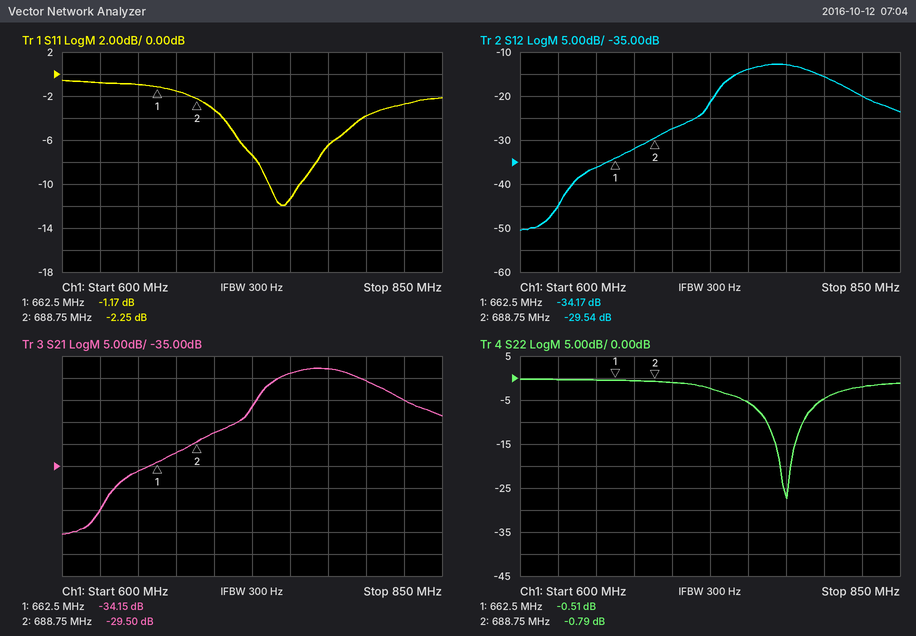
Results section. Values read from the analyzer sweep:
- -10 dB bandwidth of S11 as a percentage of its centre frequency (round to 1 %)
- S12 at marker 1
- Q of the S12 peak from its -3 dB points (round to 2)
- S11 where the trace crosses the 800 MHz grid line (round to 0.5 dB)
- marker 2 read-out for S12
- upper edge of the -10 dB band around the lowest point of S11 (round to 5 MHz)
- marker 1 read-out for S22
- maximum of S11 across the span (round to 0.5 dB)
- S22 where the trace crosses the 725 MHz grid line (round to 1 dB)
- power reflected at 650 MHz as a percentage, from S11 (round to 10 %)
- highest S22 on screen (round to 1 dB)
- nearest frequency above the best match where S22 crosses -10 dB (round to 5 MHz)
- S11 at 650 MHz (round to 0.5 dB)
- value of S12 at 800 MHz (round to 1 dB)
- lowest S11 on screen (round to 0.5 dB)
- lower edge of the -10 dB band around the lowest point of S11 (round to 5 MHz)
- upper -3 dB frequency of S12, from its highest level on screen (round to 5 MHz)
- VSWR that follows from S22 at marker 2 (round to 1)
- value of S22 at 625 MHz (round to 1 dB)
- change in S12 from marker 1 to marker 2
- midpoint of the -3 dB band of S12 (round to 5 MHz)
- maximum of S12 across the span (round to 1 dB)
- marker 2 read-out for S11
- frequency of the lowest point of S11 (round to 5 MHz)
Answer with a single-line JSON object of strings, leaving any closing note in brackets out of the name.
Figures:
{"-10 dB bandwidth of S11 as a percentage of its centre frequency": "3 %", "S12 at marker 1": "-34.17 dB", "Q of the S12 peak from its -3 dB points": "12", "S11 where the trace crosses the 800 MHz grid line": "-4.0 dB", "marker 2 read-out for S12": "-29.54 dB", "upper edge of the -10 dB band around the lowest point of S11": "755 MHz", "marker 1 read-out for S22": "-0.51 dB", "maximum of S11 across the span": "-0.5 dB", "S22 where the trace crosses the 725 MHz grid line": "-2 dB", "power reflected at 650 MHz as a percentage, from S11": "80 %", "highest S22 on screen": "0 dB", "nearest frequency above the best match where S22 crosses -10 dB": "785 MHz", "S11 at 650 MHz": "-1.0 dB", "value of S12 at 800 MHz": "-16 dB", "lowest S11 on screen": "-12.0 dB", "lower edge of the -10 dB band around the lowest point of S11": "735 MHz", "upper -3 dB frequency of S12, from its highest level on screen": "800 MHz", "VSWR that follows from S22 at marker 2": "22", "value of S22 at 625 MHz": "0 dB", "change in S12 from marker 1 to marker 2": "4.63 dB", "midpoint of the -3 dB band of S12": "770 MHz", "maximum of S12 across the span": "-13 dB", "marker 2 read-out for S11": "-2.25 dB", "frequency of the lowest point of S11": "745 MHz"}
